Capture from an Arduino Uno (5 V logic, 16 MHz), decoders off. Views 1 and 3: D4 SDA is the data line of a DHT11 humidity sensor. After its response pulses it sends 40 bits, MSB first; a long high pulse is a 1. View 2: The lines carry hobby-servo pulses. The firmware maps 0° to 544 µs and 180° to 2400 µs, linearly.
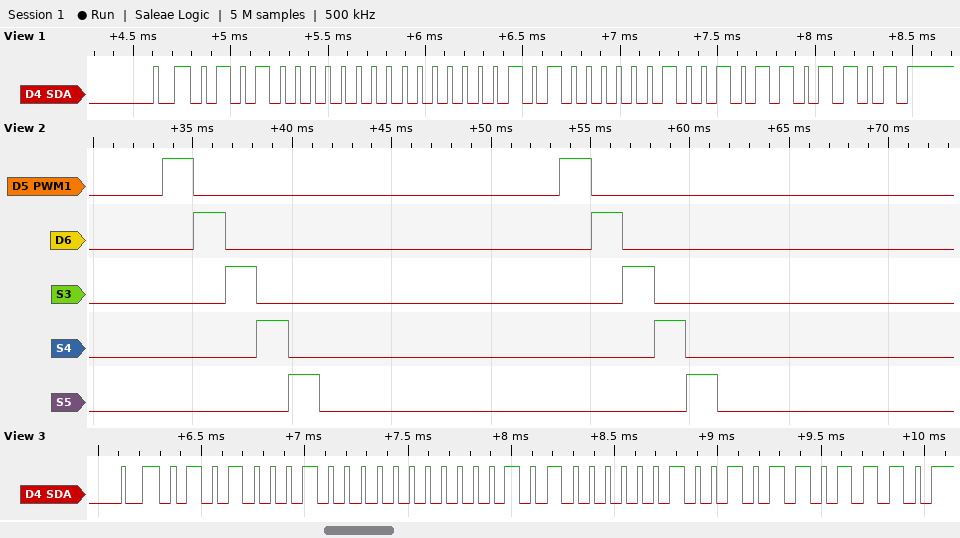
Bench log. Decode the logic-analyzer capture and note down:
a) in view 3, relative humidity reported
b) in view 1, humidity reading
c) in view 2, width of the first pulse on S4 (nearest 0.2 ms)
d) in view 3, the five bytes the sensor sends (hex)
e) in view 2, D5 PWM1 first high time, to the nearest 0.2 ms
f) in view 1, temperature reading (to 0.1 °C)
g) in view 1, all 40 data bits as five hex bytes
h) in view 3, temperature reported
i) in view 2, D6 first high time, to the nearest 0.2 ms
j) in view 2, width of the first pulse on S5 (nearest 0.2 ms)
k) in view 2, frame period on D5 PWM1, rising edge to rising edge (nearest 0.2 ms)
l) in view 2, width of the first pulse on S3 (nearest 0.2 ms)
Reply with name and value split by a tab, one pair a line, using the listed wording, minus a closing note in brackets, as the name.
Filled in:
in view 3, relative humidity reported	81 %
in view 1, humidity reading	80 %
in view 2, width of the first pulse on S4	1.6 ms
in view 3, the five bytes the sensor sends	51 00 14 09 6E
in view 2, D5 PWM1 first high time, to the nearest 0.2 ms	1.6 ms
in view 1, temperature reading	20.9 °C
in view 1, all 40 data bits as five hex bytes	50 00 14 09 6D
in view 3, temperature reported	20.9 °C
in view 2, D6 first high time, to the nearest 0.2 ms	1.6 ms
in view 2, width of the first pulse on S5	1.6 ms
in view 2, frame period on D5 PWM1, rising edge to rising edge	20.0 ms
in view 2, width of the first pulse on S3	1.6 ms
